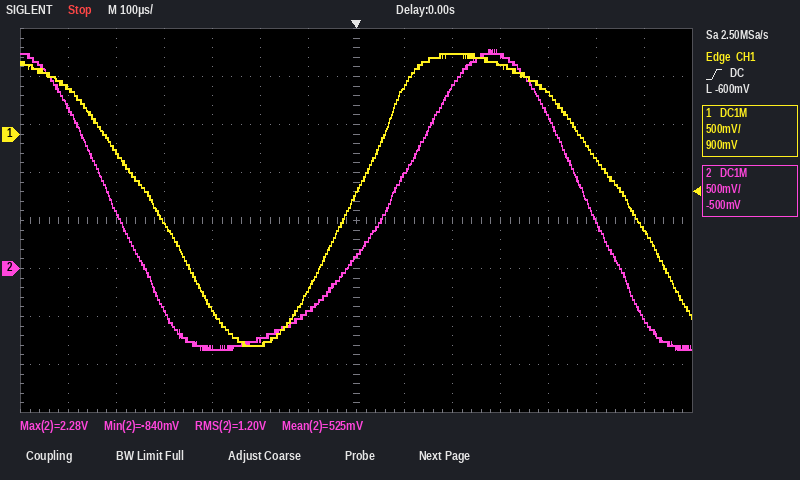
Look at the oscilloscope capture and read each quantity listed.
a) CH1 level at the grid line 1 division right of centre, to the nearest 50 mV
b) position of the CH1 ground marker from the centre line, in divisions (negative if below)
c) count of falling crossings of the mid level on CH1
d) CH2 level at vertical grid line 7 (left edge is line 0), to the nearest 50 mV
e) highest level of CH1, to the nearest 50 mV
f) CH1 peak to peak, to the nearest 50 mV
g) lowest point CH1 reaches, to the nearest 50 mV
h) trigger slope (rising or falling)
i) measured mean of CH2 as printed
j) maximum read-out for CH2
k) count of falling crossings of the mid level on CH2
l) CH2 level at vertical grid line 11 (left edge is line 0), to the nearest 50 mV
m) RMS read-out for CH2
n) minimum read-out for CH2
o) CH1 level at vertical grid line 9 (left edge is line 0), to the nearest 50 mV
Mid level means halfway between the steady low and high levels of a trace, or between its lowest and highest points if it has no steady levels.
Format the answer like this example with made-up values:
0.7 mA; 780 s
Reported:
500 mV; +1.8 div; 2; 150 mV; 850 mV; 3.05 V; -2.20 V; rising; 525 mV; 2.28 V; 2; 1.60 V; 1.20 V; -840 mV; 850 mV
